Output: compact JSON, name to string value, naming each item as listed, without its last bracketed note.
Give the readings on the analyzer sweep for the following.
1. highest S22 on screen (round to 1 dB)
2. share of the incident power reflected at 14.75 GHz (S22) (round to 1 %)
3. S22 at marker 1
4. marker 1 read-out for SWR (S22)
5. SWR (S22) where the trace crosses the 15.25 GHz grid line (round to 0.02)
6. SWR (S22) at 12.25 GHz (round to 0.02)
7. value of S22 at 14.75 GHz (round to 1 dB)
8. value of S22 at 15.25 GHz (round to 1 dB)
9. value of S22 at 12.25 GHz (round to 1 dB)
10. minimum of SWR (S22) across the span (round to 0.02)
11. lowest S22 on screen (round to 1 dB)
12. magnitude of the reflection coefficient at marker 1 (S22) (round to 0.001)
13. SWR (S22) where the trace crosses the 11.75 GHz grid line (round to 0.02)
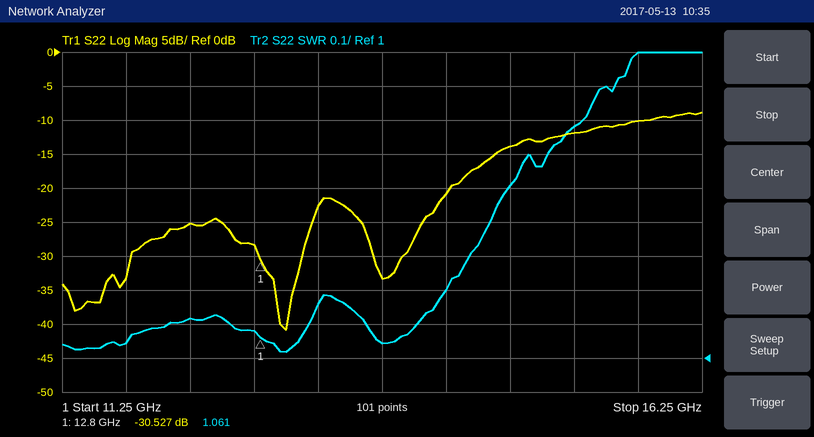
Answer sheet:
{"highest S22 on screen": "-9 dB", "share of the incident power reflected at 14.75 GHz (S22)": "4 %", "S22 at marker 1": "-30.527 dB", "marker 1 read-out for SWR": "1.061", "SWR (S22) where the trace crosses the 15.25 GHz grid line": "1.68", "SWR (S22) at 12.25 GHz": "1.12", "value of S22 at 14.75 GHz": "-14 dB", "value of S22 at 15.25 GHz": "-12 dB", "value of S22 at 12.25 GHz": "-25 dB", "minimum of SWR (S22) across the span": "1.02", "lowest S22 on screen": "-41 dB", "magnitude of the reflection coefficient at marker 1 (S22)": "0.030", "SWR (S22) where the trace crosses the 11.75 GHz grid line": "1.04"}
